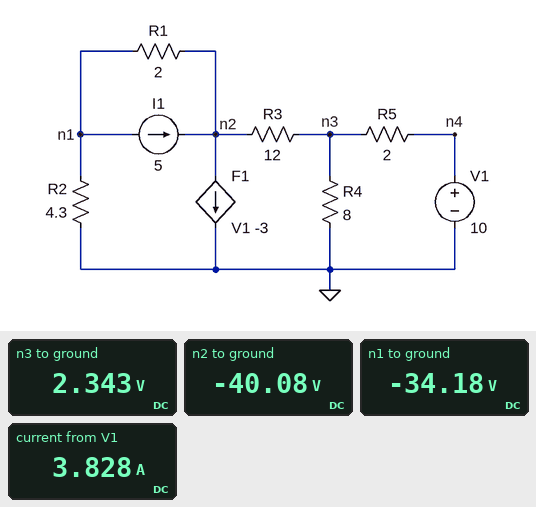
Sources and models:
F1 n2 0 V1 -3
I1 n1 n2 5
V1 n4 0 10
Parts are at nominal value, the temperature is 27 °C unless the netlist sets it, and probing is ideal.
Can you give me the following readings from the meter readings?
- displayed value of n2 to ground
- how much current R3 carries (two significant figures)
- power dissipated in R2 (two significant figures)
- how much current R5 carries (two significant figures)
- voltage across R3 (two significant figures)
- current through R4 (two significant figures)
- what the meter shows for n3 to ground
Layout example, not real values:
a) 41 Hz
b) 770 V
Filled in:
a) -40.08 V
b) 3.5 A
c) 270 W
d) 3.8 A
e) 42 V
f) 290 mA
g) 2.343 V
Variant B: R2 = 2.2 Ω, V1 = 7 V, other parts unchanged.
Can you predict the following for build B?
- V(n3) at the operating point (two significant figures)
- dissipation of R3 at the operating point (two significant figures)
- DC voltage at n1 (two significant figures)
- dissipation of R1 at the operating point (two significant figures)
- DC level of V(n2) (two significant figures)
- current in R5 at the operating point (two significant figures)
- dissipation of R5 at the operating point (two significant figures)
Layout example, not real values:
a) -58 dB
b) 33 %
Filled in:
a) 4.7 V
b) 3.9 W
c) -6.4 V
d) 8.8 W
e) -2.2 V
f) 1.2 A
g) 2.7 W
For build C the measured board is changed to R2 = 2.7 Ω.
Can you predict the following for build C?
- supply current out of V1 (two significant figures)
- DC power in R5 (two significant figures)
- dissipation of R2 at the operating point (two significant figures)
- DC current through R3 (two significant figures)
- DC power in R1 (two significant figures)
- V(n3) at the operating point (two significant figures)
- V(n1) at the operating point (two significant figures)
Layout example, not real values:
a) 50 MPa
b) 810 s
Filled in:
a) 2.4 A
b) 11 W
c) 79 W
d) 1.7 A
e) 340 mW
f) 5.2 V
g) -15 V
